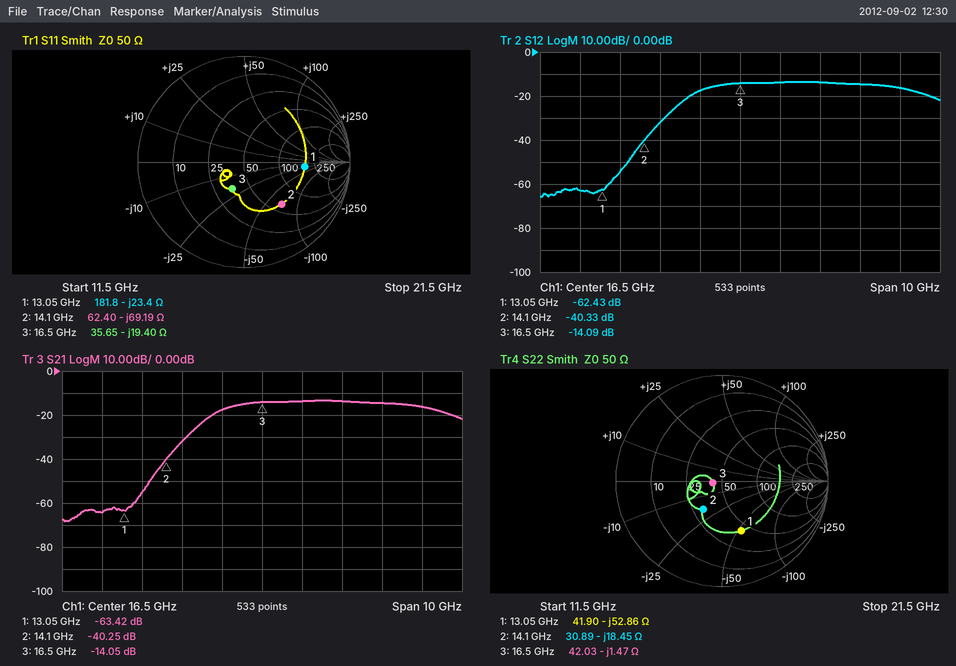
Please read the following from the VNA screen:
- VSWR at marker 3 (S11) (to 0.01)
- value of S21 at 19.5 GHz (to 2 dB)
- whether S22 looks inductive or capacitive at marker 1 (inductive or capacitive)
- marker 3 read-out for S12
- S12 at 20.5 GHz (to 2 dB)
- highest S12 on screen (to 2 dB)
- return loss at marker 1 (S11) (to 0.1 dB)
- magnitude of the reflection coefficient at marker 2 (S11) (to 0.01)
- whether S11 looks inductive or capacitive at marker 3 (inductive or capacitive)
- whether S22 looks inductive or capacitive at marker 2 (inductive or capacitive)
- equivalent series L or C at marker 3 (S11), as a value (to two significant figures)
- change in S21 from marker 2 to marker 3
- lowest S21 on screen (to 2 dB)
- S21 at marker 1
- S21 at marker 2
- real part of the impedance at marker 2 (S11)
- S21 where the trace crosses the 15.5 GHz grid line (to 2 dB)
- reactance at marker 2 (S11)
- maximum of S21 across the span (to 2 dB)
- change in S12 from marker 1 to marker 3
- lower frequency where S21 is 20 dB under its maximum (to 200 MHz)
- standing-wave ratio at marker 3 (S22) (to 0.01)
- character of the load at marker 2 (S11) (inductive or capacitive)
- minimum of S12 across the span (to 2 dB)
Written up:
1.76
-14 dB
capacitive
-14.09 dB
-16 dB
-14 dB
4.8 dB
0.53
capacitive
capacitive
500 fF
26.20 dB
-68 dB
-63.42 dB
-40.25 dB
62.40 Ω
-18 dB
-69.19 Ω
-14 dB
48.34 dB
14.4 GHz
1.19
capacitive
-66 dB
